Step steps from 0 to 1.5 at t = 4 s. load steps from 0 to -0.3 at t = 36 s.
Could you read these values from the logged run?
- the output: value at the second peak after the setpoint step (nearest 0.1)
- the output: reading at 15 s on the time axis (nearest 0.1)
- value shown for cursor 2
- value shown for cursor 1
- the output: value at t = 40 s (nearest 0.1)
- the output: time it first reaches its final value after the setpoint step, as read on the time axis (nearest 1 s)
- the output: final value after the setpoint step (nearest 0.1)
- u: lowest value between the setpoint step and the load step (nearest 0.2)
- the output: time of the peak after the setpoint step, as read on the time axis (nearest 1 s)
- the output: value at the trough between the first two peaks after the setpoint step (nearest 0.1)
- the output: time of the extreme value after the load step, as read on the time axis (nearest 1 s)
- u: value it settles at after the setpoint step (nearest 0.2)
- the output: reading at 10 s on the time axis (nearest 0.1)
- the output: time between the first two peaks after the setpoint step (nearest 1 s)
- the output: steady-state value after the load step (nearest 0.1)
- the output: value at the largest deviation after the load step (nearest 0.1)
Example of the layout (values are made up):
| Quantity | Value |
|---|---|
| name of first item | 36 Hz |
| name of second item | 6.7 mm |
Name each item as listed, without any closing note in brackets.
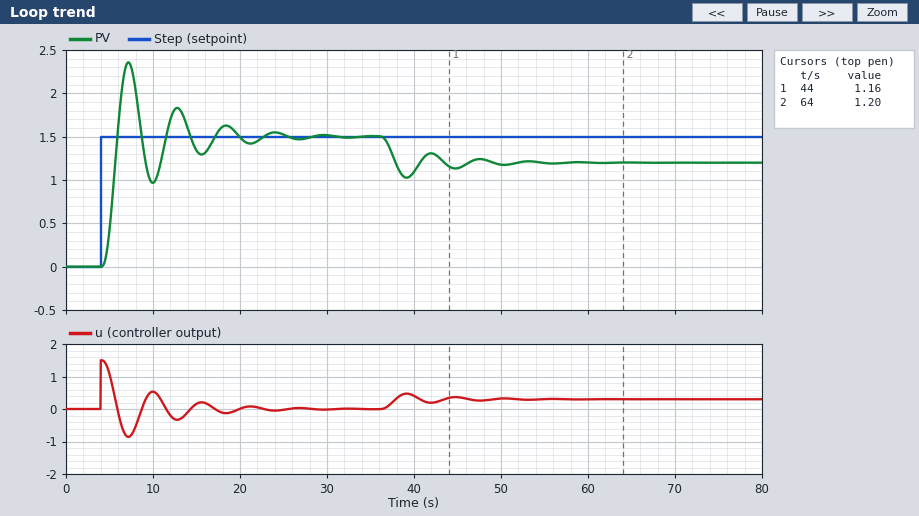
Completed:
| Quantity | Value |
|---|---|
| the output: value at the second peak after the setpoint step | 1.8 |
| the output: reading at 15 s on the time axis | 1.3 |
| value shown for cursor 2 | 1.20 |
| value shown for cursor 1 | 1.16 |
| the output: value at t = 40 s | 1.1 |
| the output: time it first reaches its final value after the setpoint step, as read on the time axis | 6 s |
| the output: final value after the setpoint step | 1.5 |
| u: lowest value between the setpoint step and the load step | -0.8 |
| the output: time of the peak after the setpoint step, as read on the time axis | 7 s |
| the output: value at the trough between the first two peaks after the setpoint step | 1.0 |
| the output: time of the extreme value after the load step, as read on the time axis | 39 s |
| u: value it settles at after the setpoint step | 0.0 |
| the output: reading at 10 s on the time axis | 1.0 |
| the output: time between the first two peaks after the setpoint step | 6 s |
| the output: steady-state value after the load step | 1.2 |
| the output: value at the largest deviation after the load step | 1.0 |
